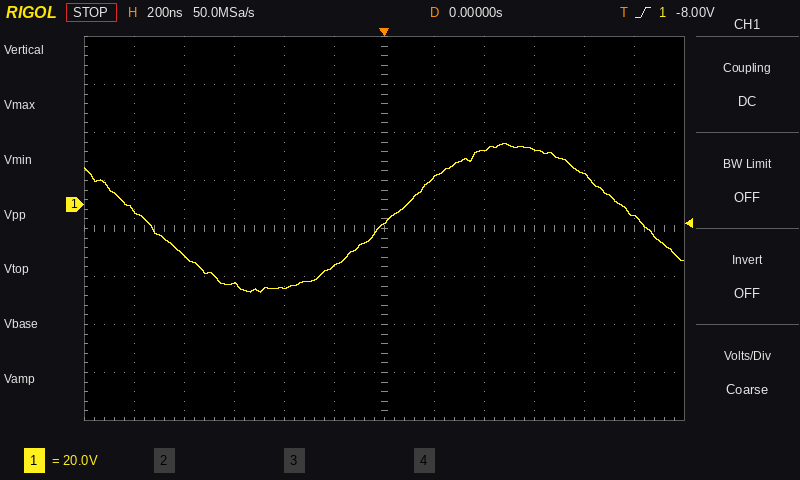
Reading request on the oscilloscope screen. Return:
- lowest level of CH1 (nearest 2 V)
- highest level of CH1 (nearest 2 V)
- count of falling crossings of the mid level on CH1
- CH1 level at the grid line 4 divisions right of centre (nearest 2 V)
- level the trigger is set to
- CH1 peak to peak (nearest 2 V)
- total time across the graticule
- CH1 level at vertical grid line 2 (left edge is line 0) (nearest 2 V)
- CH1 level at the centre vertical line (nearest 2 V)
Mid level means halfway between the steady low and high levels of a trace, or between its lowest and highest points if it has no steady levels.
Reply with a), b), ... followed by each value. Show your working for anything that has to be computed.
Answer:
a) -36 V
b) 26 V
c) 2
d) 12 V
e) -8.00 V
f) 26 V − (-36 V) = 62 V
g) 2.4 µs
h) -22 V
i) -8 V
